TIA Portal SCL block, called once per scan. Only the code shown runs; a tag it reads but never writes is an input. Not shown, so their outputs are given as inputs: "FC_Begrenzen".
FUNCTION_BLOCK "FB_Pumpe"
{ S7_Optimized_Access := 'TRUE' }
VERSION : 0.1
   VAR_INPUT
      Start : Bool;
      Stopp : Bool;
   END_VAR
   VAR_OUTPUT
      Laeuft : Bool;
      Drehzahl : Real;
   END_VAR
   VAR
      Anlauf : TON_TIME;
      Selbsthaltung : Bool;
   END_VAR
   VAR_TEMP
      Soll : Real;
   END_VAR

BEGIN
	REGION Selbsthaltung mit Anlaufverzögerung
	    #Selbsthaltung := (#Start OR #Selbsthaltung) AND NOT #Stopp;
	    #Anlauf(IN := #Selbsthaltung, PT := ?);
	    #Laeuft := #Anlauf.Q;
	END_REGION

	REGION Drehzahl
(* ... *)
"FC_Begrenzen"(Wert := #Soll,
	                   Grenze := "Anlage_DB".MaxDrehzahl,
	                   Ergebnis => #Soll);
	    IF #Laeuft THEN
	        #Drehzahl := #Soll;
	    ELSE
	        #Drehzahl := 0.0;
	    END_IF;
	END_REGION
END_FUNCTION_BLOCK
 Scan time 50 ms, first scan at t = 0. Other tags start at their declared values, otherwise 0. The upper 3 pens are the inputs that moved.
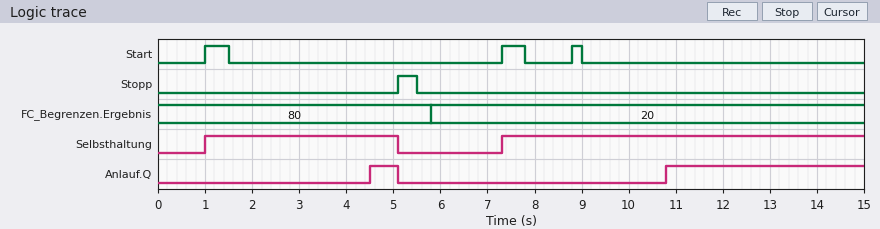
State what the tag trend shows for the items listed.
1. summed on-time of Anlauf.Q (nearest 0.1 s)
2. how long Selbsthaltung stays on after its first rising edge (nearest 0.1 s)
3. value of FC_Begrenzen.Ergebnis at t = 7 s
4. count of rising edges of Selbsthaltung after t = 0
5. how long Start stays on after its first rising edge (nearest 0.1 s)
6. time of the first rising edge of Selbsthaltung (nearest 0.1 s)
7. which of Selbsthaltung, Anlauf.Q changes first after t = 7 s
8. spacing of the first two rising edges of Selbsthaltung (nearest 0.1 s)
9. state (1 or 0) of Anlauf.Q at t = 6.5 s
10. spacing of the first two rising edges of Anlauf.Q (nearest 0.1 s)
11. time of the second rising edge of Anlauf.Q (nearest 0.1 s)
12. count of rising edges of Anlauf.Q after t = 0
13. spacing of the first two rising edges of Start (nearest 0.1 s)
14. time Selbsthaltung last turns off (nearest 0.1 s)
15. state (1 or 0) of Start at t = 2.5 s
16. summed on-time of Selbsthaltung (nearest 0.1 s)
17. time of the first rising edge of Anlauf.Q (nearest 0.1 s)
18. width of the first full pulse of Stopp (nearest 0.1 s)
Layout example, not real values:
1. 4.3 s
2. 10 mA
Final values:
1. 4.8 s
2. 4.1 s
3. 20
4. 2
5. 0.5 s
6. 1.0 s
7. Selbsthaltung
8. 6.3 s
9. 0
10. 6.3 s
11. 10.8 s
12. 2
13. 6.3 s
14. 5.1 s
15. 0
16. 11.8 s
17. 4.5 s
18. 0.4 s
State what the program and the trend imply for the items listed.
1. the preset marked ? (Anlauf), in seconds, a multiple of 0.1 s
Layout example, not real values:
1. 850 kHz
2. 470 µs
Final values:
1. 3.5 s
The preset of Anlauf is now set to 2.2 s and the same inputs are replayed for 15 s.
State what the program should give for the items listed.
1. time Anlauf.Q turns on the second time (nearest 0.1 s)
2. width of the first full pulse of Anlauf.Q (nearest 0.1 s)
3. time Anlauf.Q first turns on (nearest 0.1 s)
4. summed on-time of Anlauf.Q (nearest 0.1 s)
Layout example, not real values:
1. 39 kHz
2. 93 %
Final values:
1. 9.5 s
2. 1.9 s
3. 3.2 s
4. 7.4 s
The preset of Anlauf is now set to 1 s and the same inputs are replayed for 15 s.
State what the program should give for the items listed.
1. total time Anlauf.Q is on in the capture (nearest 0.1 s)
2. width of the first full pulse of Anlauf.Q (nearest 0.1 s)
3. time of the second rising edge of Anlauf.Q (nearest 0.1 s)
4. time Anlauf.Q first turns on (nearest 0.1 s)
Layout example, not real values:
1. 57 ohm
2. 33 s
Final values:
1. 9.8 s
2. 3.1 s
3. 8.3 s
4. 2.0 s
